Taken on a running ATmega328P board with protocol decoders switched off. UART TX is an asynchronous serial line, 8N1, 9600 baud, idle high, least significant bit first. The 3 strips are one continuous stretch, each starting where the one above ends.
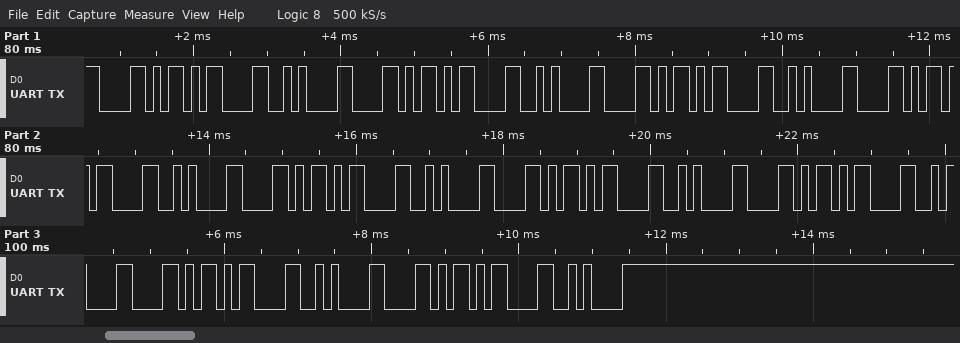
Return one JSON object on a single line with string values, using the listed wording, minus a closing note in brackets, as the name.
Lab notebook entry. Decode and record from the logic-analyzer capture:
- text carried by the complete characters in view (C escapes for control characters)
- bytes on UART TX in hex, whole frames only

{"text carried by the complete characters in view": "\"X\\r\\nX\\r\\nX\\r\\nX\\r\\nX\\r\\nX\\r\\nX\\r\\nX\\r\\nX\\r\\n\"", "bytes on UART TX in hex, whole frames only": "58 0D 0A 58 0D 0A 58 0D 0A 58 0D 0A 58 0D 0A 58 0D 0A 58 0D 0A 58 0D 0A 58 0D 0A"}
